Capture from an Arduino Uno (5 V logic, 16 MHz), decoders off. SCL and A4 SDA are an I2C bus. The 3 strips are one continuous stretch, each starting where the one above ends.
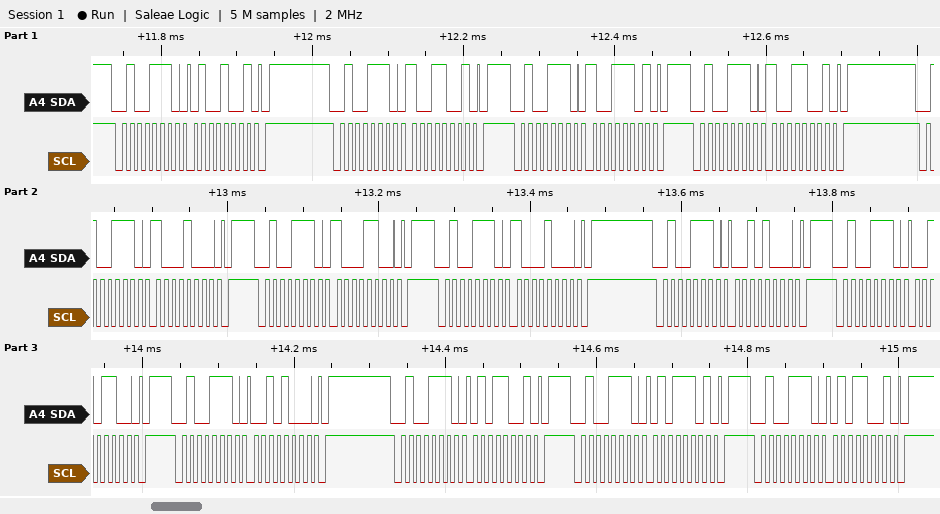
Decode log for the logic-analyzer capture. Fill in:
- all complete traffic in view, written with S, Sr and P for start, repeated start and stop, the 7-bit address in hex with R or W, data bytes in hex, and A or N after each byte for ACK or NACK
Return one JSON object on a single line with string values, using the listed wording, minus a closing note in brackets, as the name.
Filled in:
{"all complete traffic in view, written with S, Sr and P for start, repeated start and stop, the 7-bit address in hex with R or W, data bytes in hex, and A or N after each byte for ACK or NACK": "S 27W A 49 A P S 27W A 99 A P S 27W A 9D A P S 27W A 99 A P S 27W A 88 A P S 27W A 8C A P S 27W A 88 A P S 27W A 28 A P S 27W A 2C A P S 27W A 28 A P S 27W A 59 A P S 27W A 5D A P S 27W A 59 A P"}
